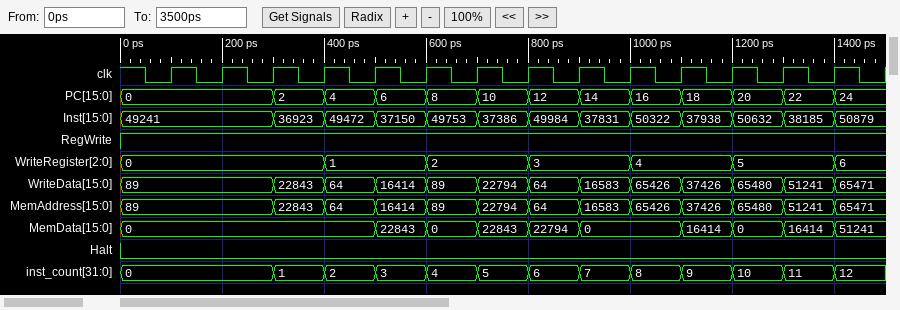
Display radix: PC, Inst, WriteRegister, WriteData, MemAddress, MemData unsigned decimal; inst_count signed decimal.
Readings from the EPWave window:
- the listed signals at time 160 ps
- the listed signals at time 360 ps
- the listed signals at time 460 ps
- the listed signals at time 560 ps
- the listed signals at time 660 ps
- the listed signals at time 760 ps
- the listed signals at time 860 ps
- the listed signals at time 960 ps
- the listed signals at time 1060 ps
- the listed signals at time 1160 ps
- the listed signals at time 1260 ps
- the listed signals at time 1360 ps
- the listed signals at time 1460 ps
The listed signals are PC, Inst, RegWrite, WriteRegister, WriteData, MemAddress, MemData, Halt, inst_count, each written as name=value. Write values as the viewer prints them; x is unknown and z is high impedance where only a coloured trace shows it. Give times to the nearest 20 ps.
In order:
PC=0, Inst=49241, RegWrite=1, WriteRegister=0, WriteData=89, MemAddress=89, MemData=0, Halt=0, inst_count=0
PC=2, Inst=36923, RegWrite=1, WriteRegister=0, WriteData=22843, MemAddress=22843, MemData=0, Halt=0, inst_count=1
PC=4, Inst=49472, RegWrite=1, WriteRegister=1, WriteData=64, MemAddress=64, MemData=0, Halt=0, inst_count=2
PC=6, Inst=37150, RegWrite=1, WriteRegister=1, WriteData=16414, MemAddress=16414, MemData=22843, Halt=0, inst_count=3
PC=8, Inst=49753, RegWrite=1, WriteRegister=2, WriteData=89, MemAddress=89, MemData=0, Halt=0, inst_count=4
PC=10, Inst=37386, RegWrite=1, WriteRegister=2, WriteData=22794, MemAddress=22794, MemData=22843, Halt=0, inst_count=5
PC=12, Inst=49984, RegWrite=1, WriteRegister=3, WriteData=64, MemAddress=64, MemData=22794, Halt=0, inst_count=6
PC=14, Inst=37831, RegWrite=1, WriteRegister=3, WriteData=16583, MemAddress=16583, MemData=0, Halt=0, inst_count=7
PC=16, Inst=50322, RegWrite=1, WriteRegister=4, WriteData=65426, MemAddress=65426, MemData=0, Halt=0, inst_count=8
PC=18, Inst=37938, RegWrite=1, WriteRegister=4, WriteData=37426, MemAddress=37426, MemData=16414, Halt=0, inst_count=9
PC=20, Inst=50632, RegWrite=1, WriteRegister=5, WriteData=65480, MemAddress=65480, MemData=0, Halt=0, inst_count=10
PC=22, Inst=38185, RegWrite=1, WriteRegister=5, WriteData=51241, MemAddress=51241, MemData=16414, Halt=0, inst_count=11
PC=24, Inst=50879, RegWrite=1, WriteRegister=6, WriteData=65471, MemAddress=65471, MemData=51241, Halt=0, inst_count=12
